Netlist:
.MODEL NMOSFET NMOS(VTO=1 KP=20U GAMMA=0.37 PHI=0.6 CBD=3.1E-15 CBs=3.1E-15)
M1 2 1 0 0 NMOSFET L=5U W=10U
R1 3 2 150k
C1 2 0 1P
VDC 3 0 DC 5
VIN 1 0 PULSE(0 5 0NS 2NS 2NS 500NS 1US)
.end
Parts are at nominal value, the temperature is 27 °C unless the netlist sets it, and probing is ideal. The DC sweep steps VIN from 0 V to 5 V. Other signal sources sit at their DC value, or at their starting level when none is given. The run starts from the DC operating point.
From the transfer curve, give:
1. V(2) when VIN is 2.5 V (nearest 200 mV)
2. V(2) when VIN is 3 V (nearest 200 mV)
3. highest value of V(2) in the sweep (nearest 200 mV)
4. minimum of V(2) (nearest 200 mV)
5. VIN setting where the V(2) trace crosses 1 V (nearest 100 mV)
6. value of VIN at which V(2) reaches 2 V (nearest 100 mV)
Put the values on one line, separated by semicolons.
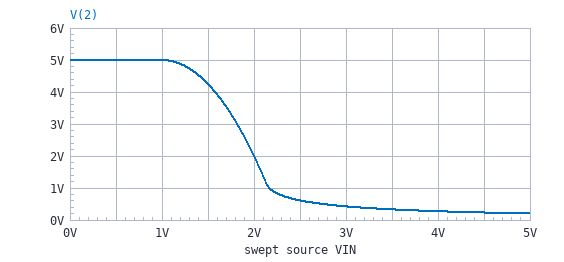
600 mV; 400 mV; 5.0 V; 200 mV; 2.2 V; 2.0 V
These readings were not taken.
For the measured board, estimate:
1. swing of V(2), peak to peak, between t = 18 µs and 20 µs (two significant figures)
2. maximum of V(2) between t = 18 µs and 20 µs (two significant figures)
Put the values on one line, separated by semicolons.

4.6 V; 4.8 V
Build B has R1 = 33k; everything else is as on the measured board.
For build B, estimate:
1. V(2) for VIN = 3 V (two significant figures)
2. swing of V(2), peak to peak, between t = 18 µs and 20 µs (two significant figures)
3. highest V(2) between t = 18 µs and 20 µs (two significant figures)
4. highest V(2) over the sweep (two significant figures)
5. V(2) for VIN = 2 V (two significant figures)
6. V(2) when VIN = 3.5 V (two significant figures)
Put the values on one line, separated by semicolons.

2.4 V; 4.1 V; 5.0 V; 5.0 V; 4.3 V; 1.5 V
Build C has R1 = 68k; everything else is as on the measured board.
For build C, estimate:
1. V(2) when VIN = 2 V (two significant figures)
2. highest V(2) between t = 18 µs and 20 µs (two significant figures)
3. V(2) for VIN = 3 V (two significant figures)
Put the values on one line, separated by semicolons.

3.6 V; 5.0 V; 980 mV
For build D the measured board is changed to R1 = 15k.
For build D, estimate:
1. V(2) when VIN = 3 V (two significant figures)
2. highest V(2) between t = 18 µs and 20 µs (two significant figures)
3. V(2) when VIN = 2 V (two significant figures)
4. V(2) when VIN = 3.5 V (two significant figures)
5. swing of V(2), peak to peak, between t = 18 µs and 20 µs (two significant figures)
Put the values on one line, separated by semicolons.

3.8 V; 5.0 V; 4.7 V; 3.1 V; 3.3 V
